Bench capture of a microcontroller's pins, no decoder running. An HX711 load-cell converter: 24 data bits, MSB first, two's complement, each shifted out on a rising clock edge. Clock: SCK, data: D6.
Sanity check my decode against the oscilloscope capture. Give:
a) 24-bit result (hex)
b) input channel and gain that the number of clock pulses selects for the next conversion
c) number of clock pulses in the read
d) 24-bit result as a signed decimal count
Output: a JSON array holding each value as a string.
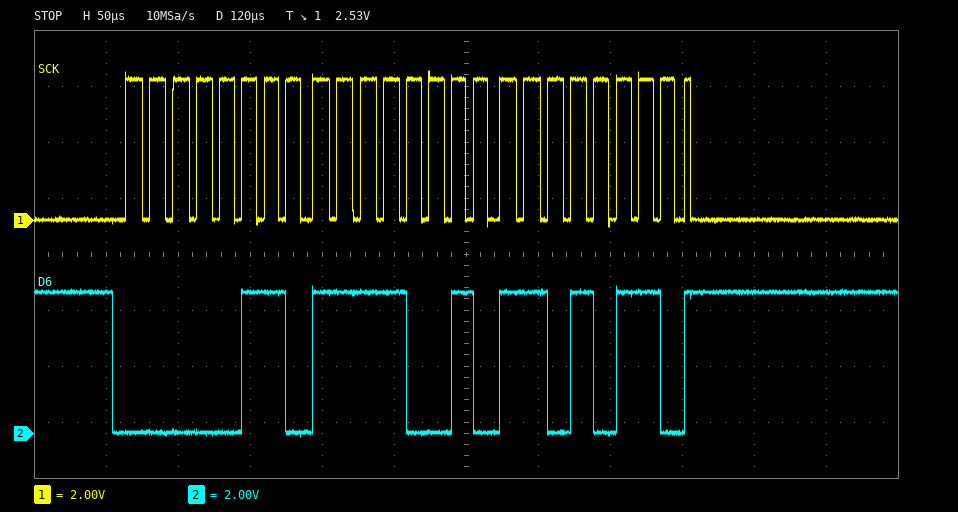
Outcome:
["0x06F2D6", "channel A, gain 128", "25", "455382"]
